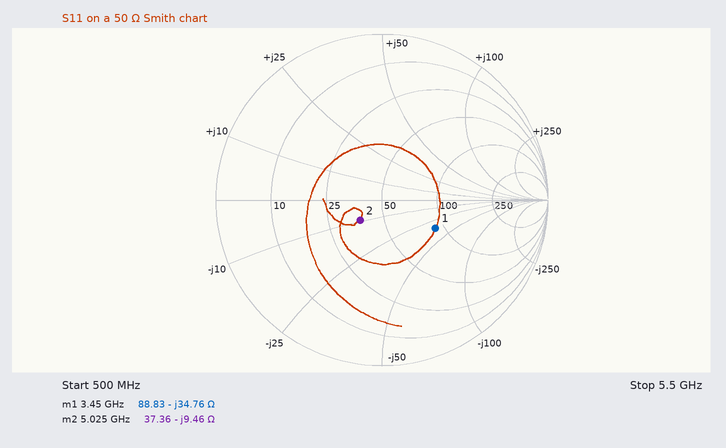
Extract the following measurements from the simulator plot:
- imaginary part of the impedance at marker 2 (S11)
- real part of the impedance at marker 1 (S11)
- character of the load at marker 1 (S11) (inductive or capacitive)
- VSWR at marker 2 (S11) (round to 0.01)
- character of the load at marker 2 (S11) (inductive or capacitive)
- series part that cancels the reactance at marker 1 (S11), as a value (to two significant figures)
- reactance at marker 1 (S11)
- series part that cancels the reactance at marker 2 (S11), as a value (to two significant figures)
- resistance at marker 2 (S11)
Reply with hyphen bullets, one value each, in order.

- -9.46 Ω
- 88.83 Ω
- capacitive
- 1.44
- capacitive
- 1.6 nH
- -34.76 Ω
- 300 pH
- 37.36 Ω
